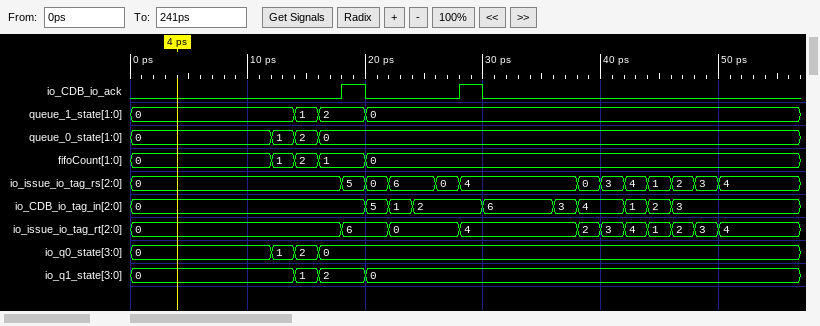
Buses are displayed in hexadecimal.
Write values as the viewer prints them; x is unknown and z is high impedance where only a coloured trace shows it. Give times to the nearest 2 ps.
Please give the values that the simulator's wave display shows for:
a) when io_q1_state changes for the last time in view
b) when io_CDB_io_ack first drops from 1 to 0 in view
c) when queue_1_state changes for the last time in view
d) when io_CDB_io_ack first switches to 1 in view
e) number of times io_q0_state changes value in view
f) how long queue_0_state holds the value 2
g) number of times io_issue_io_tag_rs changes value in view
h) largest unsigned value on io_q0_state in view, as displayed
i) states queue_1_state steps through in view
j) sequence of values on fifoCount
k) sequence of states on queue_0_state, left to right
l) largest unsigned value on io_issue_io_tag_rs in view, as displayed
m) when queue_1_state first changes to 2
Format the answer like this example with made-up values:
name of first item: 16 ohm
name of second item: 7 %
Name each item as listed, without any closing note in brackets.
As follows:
when io_q1_state changes for the last time in view: 20 ps
when io_CDB_io_ack first drops from 1 to 0 in view: 20 ps
when queue_1_state changes for the last time in view: 20 ps
when io_CDB_io_ack first switches to 1 in view: 18 ps
number of times io_q0_state changes value in view: 3
how long queue_0_state holds the value 2: 2 ps
number of times io_issue_io_tag_rs changes value in view: 12
largest unsigned value on io_q0_state in view, as displayed: 2
states queue_1_state steps through in view: 0, 1, 2, 0
sequence of values on fifoCount: 0, 1, 2, 1, 0
sequence of states on queue_0_state, left to right: 0, 1, 2, 0
largest unsigned value on io_issue_io_tag_rs in view, as displayed: 6
when queue_1_state first changes to 2: 16 ps
